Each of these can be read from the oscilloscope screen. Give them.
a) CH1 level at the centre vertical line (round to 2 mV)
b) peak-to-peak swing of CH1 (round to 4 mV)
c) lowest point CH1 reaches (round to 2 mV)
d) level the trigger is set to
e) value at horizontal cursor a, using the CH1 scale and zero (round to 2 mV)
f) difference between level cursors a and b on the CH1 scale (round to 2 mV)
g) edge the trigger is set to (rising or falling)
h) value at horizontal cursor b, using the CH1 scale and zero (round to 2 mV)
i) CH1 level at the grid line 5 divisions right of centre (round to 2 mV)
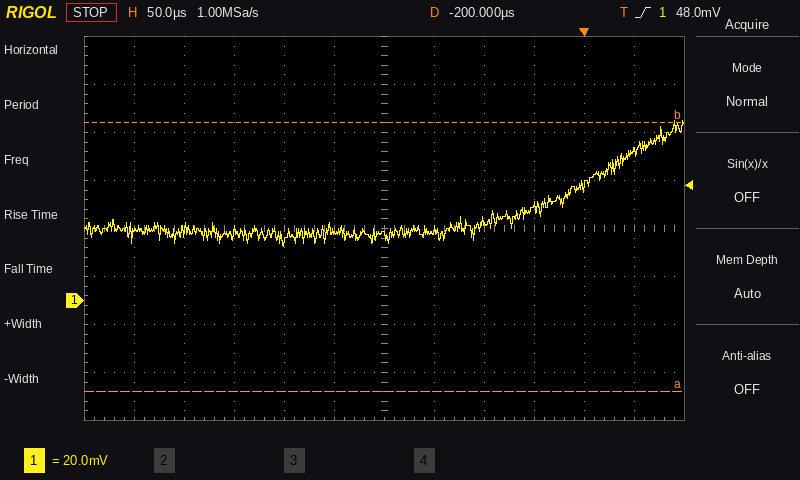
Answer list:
26 mV
52 mV
22 mV
48.0 mV
-38 mV
112 mV
rising
74 mV
62 mV
